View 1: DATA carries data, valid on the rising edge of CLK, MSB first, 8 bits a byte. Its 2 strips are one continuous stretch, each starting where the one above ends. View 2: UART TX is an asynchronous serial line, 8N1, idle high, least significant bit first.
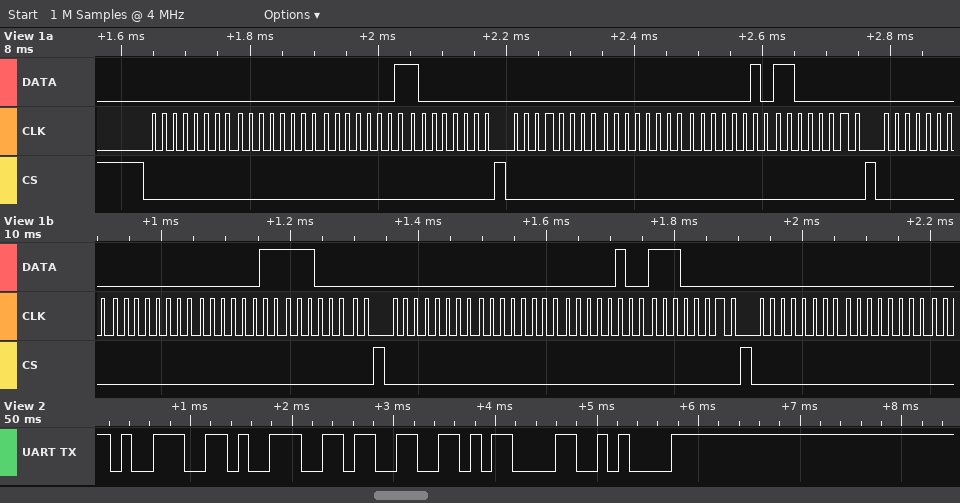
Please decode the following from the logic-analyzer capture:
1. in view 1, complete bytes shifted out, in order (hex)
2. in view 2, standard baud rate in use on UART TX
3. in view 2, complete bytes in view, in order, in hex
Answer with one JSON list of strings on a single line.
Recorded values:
["00 00 01 80 00 00 02 C0 00 00 03 E0 00 00 04 E0 00 00", "9600 baud", "39 39 33 0D 0A"]
